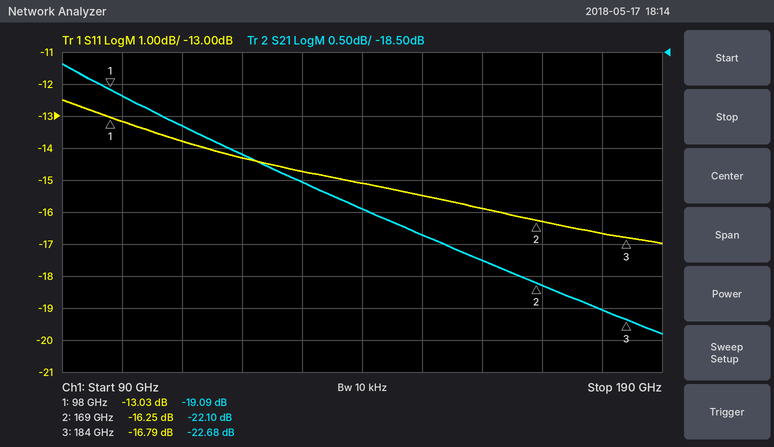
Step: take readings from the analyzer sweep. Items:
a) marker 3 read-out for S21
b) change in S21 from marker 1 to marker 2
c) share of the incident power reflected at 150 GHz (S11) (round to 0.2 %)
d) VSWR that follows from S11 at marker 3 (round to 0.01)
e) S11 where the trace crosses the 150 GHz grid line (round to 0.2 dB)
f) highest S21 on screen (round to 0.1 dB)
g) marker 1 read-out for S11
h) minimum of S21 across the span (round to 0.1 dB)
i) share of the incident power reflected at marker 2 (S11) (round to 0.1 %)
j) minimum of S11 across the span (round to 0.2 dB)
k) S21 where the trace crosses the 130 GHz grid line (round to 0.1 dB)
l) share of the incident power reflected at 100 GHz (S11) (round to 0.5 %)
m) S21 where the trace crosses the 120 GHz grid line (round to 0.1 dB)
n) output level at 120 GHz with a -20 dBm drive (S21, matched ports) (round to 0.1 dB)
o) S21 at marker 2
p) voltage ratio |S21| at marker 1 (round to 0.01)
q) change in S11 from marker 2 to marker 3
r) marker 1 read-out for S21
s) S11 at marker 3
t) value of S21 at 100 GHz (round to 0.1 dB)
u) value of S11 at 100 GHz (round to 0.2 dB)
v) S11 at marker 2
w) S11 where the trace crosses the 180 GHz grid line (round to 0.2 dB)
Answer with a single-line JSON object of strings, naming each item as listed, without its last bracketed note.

{"marker 3 read-out for S21": "-22.68 dB", "change in S21 from marker 1 to marker 2": "-3.01 dB", "share of the incident power reflected at 150 GHz (S11)": "2.8 %", "VSWR that follows from S11 at marker 3": "1.34", "S11 where the trace crosses the 150 GHz grid line": "-15.4 dB", "highest S21 on screen": "-18.7 dB", "marker 1 read-out for S11": "-13.03 dB", "minimum of S21 across the span": "-22.9 dB", "share of the incident power reflected at marker 2 (S11)": "2.4 %", "minimum of S11 across the span": "-17.0 dB", "S21 where the trace crosses the 130 GHz grid line": "-20.5 dB", "share of the incident power reflected at 100 GHz (S11)": "5.0 %", "S21 where the trace crosses the 120 GHz grid line": "-20.1 dB", "output level at 120 GHz with a -20 dBm drive (S21, matched ports)": "-40.1 dBm", "S21 at marker 2": "-22.10 dB", "voltage ratio |S21| at marker 1": "0.11", "change in S11 from marker 2 to marker 3": "-0.54 dB", "marker 1 read-out for S21": "-19.09 dB", "S11 at marker 3": "-16.79 dB", "value of S21 at 100 GHz": "-19.2 dB", "value of S11 at 100 GHz": "-13.2 dB", "S11 at marker 2": "-16.25 dB", "S11 where the trace crosses the 180 GHz grid line": "-16.6 dB"}
